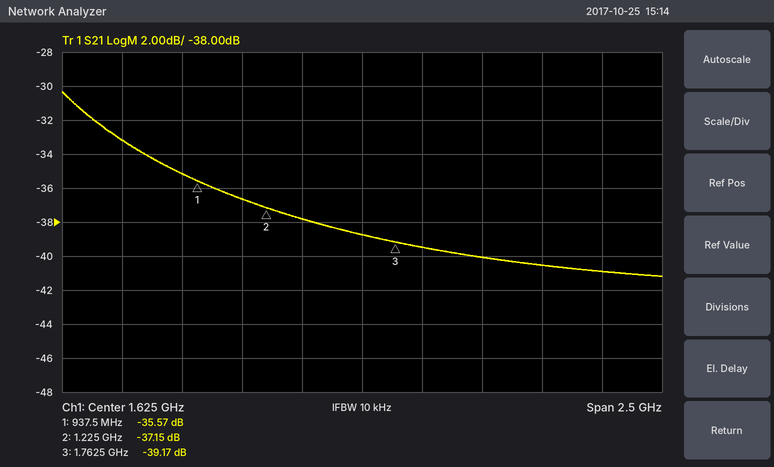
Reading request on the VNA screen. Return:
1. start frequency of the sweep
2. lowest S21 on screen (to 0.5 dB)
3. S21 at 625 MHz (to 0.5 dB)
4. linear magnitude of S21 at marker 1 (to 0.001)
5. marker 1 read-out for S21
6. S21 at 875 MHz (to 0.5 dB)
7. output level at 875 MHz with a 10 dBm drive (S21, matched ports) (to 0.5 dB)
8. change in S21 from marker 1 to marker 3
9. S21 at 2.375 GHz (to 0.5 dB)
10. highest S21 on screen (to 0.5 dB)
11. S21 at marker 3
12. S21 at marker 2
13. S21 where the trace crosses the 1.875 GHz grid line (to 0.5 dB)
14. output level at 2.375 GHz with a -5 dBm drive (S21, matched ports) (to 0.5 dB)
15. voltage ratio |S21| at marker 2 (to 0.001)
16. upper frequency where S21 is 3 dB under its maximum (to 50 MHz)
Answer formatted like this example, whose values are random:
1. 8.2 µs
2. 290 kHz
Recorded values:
1. 375 MHz
2. -41.0 dB
3. -33.0 dB
4. 0.017
5. -35.57 dB
6. -35.0 dB
7. -25.0 dBm
8. -3.60 dB
9. -40.5 dB
10. -30.5 dB
11. -39.17 dB
12. -37.15 dB
13. -39.5 dB
14. -45.5 dBm
15. 0.014
16. 650 MHz
